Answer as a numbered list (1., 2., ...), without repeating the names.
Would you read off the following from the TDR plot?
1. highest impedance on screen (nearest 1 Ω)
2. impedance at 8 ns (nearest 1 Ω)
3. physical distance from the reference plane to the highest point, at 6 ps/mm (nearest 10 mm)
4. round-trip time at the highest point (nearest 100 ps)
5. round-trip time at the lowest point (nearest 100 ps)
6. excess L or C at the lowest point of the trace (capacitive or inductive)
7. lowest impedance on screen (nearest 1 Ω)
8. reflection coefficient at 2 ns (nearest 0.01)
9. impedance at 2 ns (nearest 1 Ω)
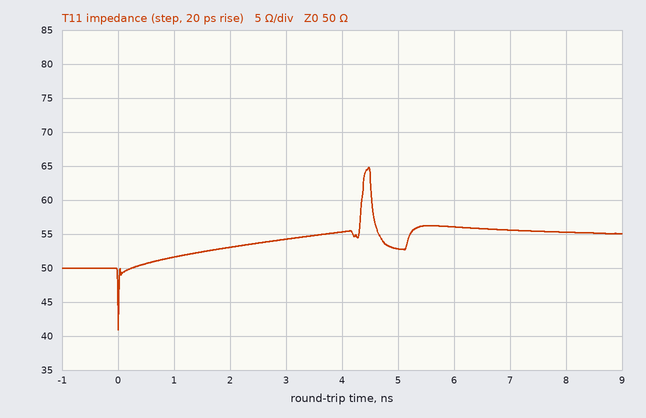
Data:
1. 65 Ω
2. 55 Ω
3. 370 mm
4. 4.5 ns
5. 0.0 ns
6. capacitive
7. 41 Ω
8. +0.03
9. 53 Ω
